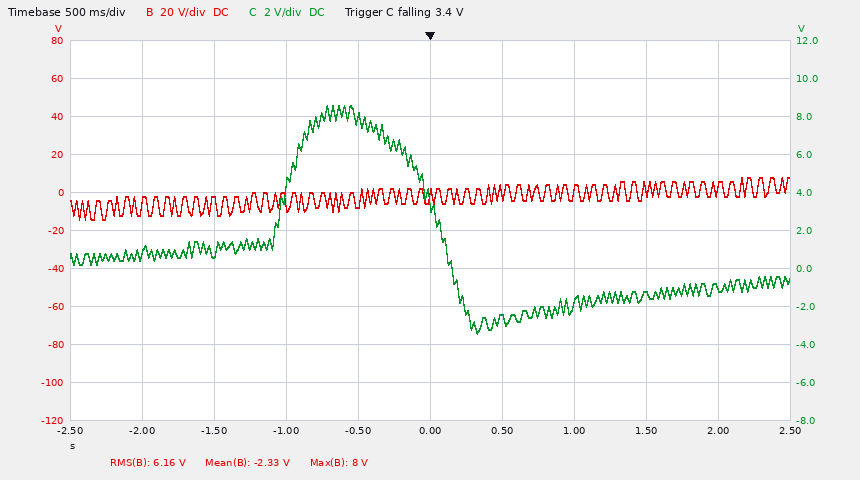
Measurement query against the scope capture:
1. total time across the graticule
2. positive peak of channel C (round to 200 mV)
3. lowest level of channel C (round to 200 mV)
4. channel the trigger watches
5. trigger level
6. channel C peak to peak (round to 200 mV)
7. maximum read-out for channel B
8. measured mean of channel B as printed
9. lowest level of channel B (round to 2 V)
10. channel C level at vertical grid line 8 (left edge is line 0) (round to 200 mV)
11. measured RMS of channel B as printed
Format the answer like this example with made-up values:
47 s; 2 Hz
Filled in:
5 s; 8.6 V; -3.4 V; channel C; 3.4 V; 12.0 V; 8 V; -2.33 V; -14 V; -1.4 V; 6.16 V
